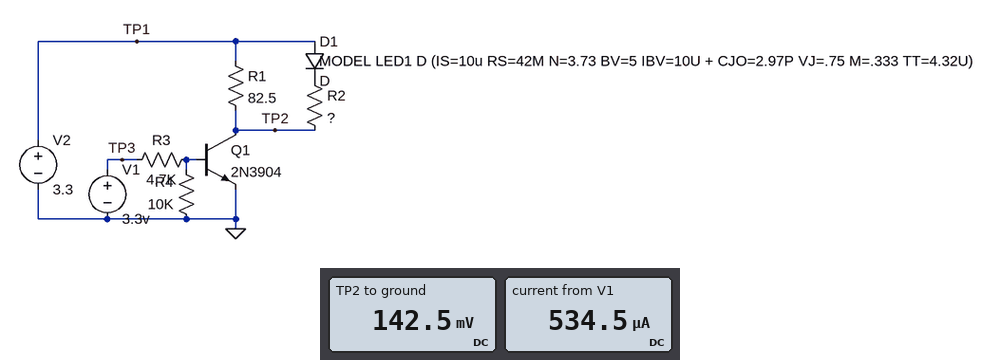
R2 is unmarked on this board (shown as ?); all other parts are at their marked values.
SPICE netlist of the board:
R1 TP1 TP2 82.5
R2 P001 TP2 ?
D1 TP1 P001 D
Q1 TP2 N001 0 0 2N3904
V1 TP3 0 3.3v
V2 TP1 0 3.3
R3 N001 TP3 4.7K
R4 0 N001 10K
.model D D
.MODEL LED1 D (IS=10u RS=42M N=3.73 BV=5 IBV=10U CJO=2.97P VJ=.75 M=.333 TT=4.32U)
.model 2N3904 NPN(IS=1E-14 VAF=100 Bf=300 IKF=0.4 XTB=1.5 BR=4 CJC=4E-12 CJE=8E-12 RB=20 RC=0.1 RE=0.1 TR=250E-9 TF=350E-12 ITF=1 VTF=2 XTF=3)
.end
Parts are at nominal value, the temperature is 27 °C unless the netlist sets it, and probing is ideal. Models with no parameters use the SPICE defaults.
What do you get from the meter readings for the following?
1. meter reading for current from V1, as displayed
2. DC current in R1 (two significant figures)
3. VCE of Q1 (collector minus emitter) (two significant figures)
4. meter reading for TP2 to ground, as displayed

534.5 µA
38 mA
140 mV
142.5 mV
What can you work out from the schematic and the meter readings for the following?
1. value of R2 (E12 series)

68 Ω
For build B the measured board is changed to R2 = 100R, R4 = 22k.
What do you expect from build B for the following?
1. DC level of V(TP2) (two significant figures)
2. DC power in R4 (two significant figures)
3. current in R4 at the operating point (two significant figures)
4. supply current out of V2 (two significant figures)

120 mV
28 µW
36 µA
63 mA
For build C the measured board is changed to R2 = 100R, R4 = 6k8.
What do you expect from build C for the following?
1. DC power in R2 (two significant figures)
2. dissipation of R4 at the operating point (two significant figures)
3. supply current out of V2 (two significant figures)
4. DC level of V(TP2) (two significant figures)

59 mW
90 µW
63 mA
130 mV
